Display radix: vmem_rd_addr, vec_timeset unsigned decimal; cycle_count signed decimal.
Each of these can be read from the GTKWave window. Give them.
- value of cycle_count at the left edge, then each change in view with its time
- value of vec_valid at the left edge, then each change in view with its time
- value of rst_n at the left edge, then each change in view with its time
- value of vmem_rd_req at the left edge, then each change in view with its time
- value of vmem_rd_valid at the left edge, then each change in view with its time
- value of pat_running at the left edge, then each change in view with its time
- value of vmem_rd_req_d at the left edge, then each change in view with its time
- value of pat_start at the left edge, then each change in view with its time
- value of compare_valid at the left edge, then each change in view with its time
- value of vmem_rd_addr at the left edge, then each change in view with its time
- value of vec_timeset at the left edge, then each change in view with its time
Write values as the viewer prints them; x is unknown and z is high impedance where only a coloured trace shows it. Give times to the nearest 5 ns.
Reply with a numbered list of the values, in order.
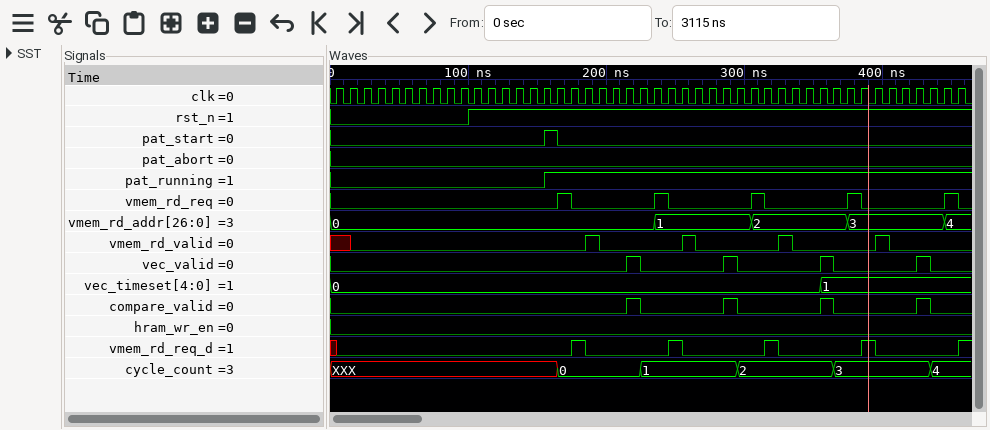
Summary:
1. XXX, 0 at 165 ns, 1 at 225 ns, 2 at 295 ns, 3 at 365 ns, 4 at 435 ns
2. 0, 1 at 215 ns, 0 at 225 ns, 1 at 285 ns, 0 at 295 ns, 1 at 355 ns, 0 at 365 ns, 1 at 425 ns, 0 at 435 ns
3. 0, 1 at 100 ns
4. 0, 1 at 165 ns, 0 at 175 ns, 1 at 235 ns, 0 at 245 ns, 1 at 305 ns, 0 at 315 ns, 1 at 375 ns, 0 at 385 ns, 1 at 445 ns, 0 at 455 ns
5. x, 0 at 15 ns, 1 at 185 ns, 0 at 195 ns, 1 at 255 ns, 0 at 265 ns, 1 at 325 ns, 0 at 335 ns, 1 at 395 ns, 0 at 405 ns
6. 0, 1 at 155 ns
7. x, 0 at 5 ns, 1 at 175 ns, 0 at 185 ns, 1 at 245 ns, 0 at 255 ns, 1 at 315 ns, 0 at 325 ns, 1 at 385 ns, 0 at 395 ns, 1 at 455 ns
8. 0, 1 at 155 ns, 0 at 165 ns
9. 0, 1 at 215 ns, 0 at 225 ns, 1 at 285 ns, 0 at 295 ns, 1 at 355 ns, 0 at 365 ns, 1 at 425 ns, 0 at 435 ns
10. 0, 1 at 235 ns, 2 at 305 ns, 3 at 375 ns, 4 at 445 ns
11. 0, 1 at 355 ns
